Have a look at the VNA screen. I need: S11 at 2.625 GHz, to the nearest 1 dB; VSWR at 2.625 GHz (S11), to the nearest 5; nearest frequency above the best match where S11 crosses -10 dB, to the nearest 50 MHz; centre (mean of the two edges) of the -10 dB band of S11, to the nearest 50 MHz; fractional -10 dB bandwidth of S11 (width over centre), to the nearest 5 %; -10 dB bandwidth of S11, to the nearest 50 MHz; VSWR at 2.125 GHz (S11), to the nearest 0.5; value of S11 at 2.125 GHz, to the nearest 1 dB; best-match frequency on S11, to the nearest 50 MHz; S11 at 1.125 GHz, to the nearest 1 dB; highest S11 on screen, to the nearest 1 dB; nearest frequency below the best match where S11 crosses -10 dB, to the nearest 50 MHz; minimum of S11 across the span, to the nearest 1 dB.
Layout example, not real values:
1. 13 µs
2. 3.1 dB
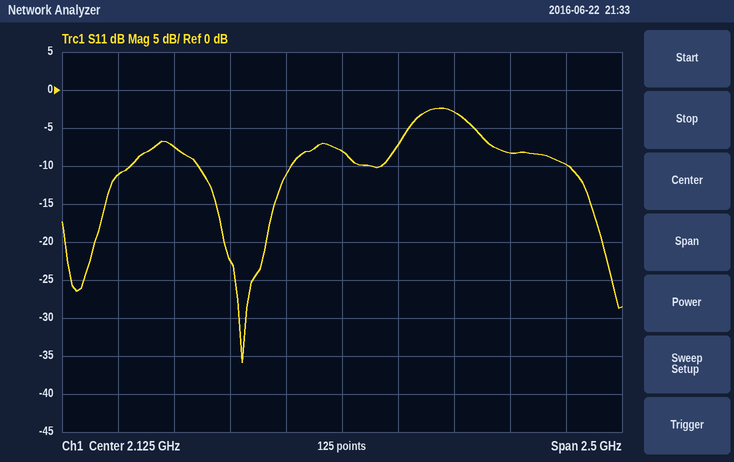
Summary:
1. -3 dB
2. 5
3. 1.90 GHz
4. 1.70 GHz
5. 25 %
6. 400 MHz
7. 2.5
8. -8 dB
9. 1.70 GHz
10. -11 dB
11. -2 dB
12. 1.50 GHz
13. -36 dB
